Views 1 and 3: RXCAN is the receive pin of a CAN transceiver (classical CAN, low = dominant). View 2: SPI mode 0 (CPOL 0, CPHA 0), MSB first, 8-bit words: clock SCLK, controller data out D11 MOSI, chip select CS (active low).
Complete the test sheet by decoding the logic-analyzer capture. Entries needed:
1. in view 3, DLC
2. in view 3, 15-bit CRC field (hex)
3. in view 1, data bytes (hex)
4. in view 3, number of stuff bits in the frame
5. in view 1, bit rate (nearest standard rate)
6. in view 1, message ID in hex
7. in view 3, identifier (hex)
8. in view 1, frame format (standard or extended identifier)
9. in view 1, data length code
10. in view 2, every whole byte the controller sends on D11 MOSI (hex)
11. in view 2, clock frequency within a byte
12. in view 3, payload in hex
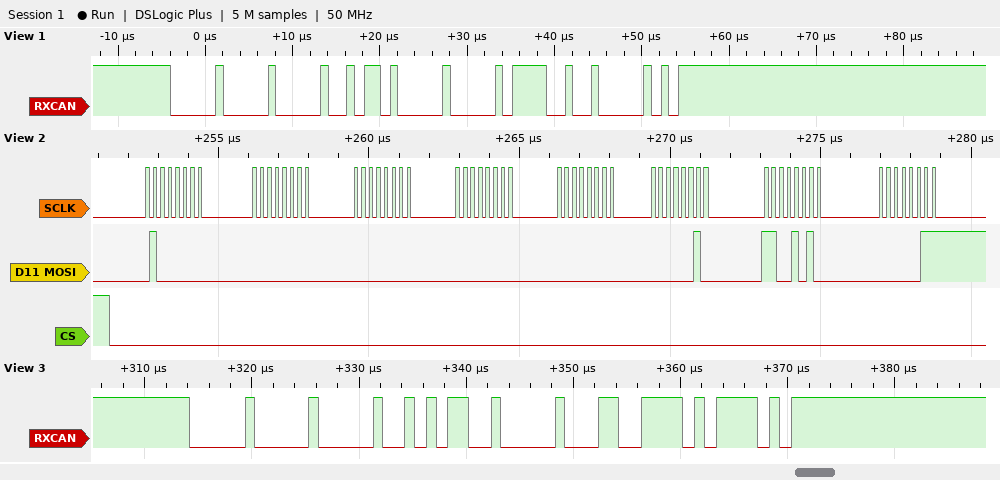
2
0x4F5E
D0 01
4
1000 kbit/s
0x000
0x000
standard
2
40 00 00 00 00 02 CA 03
4 MHz
B2 01
